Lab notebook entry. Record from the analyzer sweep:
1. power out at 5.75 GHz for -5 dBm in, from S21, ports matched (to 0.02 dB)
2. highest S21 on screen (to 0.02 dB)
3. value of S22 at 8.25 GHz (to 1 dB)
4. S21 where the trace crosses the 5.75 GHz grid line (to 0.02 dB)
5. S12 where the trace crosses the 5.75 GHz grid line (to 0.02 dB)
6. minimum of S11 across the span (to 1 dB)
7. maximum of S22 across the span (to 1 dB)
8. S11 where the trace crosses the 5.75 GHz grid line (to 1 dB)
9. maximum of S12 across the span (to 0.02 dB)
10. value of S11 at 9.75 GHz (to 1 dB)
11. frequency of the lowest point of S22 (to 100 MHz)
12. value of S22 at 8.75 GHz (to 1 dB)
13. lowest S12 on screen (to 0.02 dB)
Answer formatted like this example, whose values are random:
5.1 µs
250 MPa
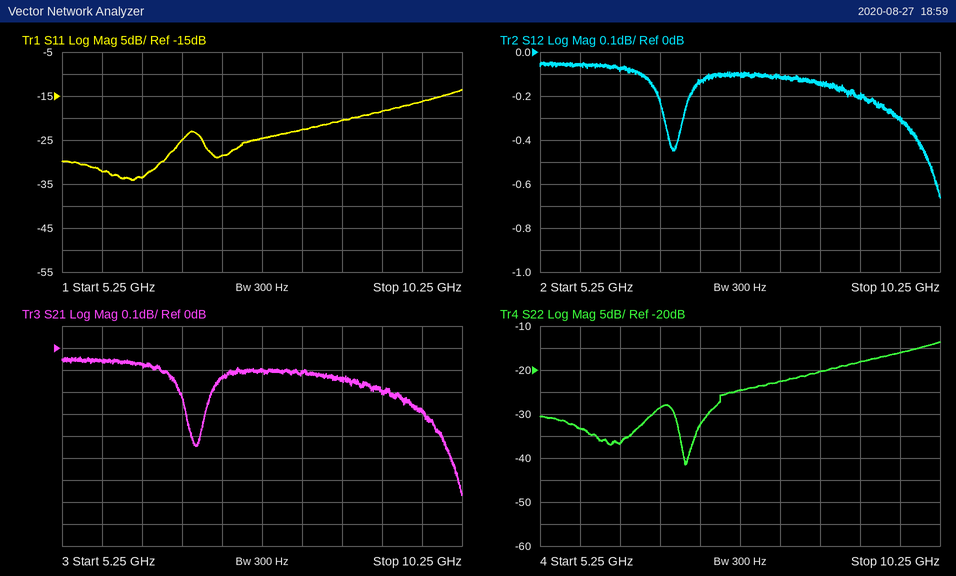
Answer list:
-5.06 dBm
-0.04 dB
-23 dB
-0.06 dB
-0.06 dB
-34 dB
-14 dB
-32 dB
-0.04 dB
-16 dB
7.1 GHz
-20 dB
-0.66 dB
